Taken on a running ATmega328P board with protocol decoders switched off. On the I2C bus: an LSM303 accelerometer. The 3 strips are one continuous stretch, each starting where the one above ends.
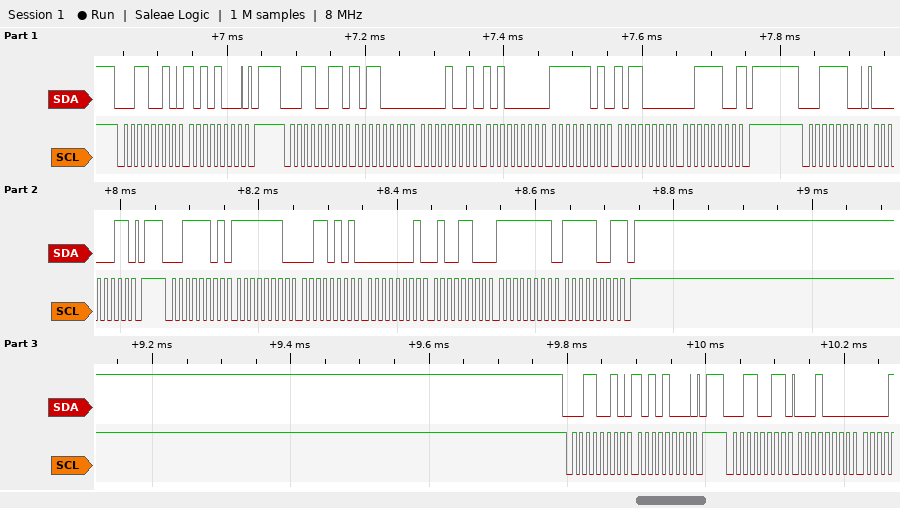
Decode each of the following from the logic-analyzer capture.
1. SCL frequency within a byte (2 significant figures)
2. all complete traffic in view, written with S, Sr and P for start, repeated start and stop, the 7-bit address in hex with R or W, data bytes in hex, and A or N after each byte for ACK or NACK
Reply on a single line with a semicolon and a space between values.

100 kHz; S 19W A A8 A P S 19R A B0 A 09 A A0 A FD A B0 A 3C N P S 1EW A 03 A P S 1ER A FE A 35 A 01 A 4C A FF A F9 N P S 19W A A8 A P S 19R A 10 A
